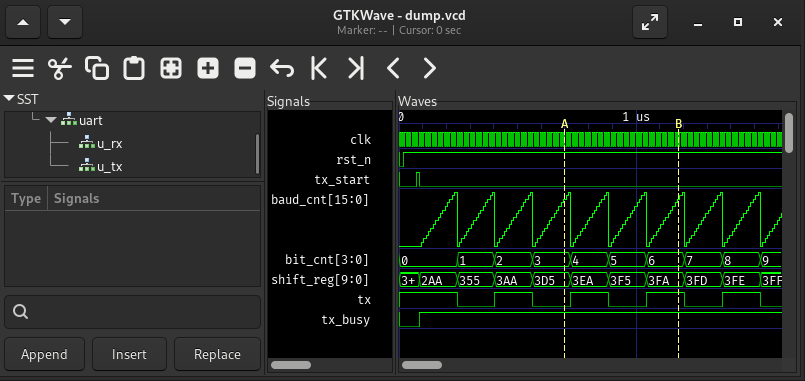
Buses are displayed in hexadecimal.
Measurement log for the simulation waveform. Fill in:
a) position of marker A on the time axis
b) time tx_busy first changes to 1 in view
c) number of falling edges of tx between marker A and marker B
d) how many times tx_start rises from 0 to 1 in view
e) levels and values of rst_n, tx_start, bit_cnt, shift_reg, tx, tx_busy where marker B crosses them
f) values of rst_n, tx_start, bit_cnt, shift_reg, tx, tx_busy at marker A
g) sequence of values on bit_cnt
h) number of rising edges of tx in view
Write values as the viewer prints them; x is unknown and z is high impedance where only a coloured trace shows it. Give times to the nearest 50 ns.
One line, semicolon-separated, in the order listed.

700 ns; 100 ns; 1; 1; rst_n=1, tx_start=0, bit_cnt=6, shift_reg=3FA, tx=1, tx_busy=1; rst_n=1, tx_start=0, bit_cnt=3, shift_reg=3D5, tx=0, tx_busy=1; 0, 1, 2, 3, 4, 5, 6, 7, 8, 9; 4
